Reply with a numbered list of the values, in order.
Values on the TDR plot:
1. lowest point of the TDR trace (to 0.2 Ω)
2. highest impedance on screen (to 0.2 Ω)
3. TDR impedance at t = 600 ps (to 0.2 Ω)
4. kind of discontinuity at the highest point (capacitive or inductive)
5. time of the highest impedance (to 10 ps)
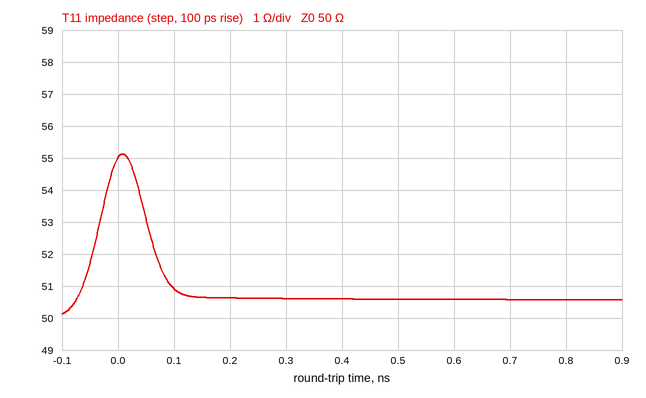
1. 50.2 Ω
2. 55.2 Ω
3. 50.6 Ω
4. inductive
5. 10 ps
